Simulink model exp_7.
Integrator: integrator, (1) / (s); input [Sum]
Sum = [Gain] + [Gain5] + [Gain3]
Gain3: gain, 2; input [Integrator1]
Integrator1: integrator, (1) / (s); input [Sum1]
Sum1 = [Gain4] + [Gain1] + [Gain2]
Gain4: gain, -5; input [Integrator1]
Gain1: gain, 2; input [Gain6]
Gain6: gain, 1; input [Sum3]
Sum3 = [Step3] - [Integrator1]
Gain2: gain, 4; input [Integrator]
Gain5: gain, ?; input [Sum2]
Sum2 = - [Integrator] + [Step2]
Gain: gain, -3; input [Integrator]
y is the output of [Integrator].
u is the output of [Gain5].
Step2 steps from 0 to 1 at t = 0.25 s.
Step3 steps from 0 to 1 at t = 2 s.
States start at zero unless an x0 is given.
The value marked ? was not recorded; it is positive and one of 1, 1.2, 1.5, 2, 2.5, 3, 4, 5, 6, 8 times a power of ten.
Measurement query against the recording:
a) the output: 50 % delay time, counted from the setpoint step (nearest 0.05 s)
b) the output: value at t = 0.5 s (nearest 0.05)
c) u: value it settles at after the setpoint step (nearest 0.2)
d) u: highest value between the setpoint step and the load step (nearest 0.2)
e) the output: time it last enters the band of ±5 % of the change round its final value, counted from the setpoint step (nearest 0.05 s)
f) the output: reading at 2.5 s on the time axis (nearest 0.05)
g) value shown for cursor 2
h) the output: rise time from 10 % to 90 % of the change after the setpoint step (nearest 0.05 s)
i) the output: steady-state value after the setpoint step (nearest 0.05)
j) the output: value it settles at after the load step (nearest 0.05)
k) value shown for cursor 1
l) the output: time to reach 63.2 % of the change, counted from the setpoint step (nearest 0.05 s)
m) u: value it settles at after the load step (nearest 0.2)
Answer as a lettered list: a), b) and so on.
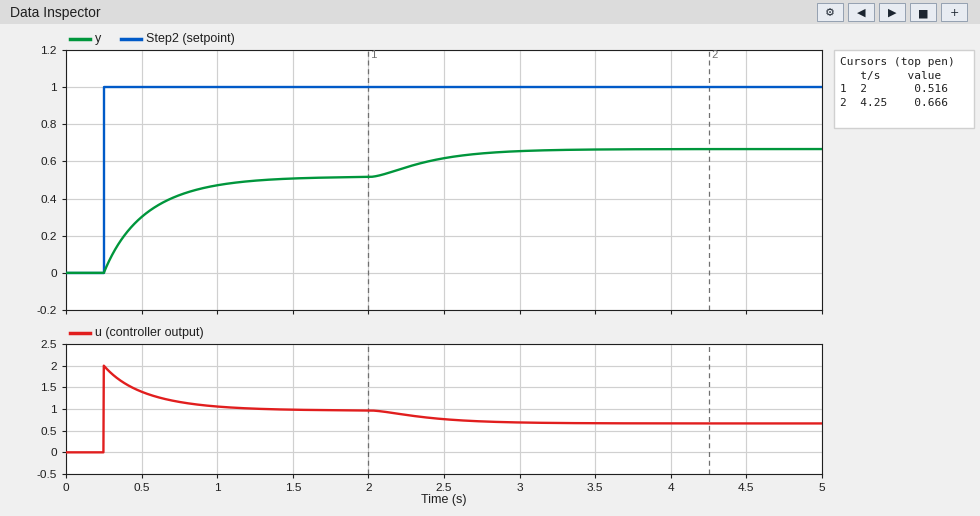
a) 0.20 s
b) 0.30
c) 1.0
d) 2.0
e) 0.95 s
f) 0.60
g) 0.666
h) 0.70 s
i) 0.50
j) 0.65
k) 0.516
l) 0.30 s
m) 0.6
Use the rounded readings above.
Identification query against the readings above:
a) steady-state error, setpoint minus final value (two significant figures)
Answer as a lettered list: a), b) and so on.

a) 0.50
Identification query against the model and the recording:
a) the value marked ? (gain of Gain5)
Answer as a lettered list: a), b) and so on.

a) 2
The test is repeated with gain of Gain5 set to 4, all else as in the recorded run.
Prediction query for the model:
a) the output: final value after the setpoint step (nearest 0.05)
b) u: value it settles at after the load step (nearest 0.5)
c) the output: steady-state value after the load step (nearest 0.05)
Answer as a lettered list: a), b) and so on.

a) 0.70
b) 1.0
c) 0.80
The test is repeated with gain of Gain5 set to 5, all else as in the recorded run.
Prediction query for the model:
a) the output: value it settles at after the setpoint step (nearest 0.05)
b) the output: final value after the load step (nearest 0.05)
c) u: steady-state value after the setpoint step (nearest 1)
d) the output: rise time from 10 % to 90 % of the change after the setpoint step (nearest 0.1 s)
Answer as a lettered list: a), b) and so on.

a) 0.75
b) 0.80
c) 1
d) 0.4 s
